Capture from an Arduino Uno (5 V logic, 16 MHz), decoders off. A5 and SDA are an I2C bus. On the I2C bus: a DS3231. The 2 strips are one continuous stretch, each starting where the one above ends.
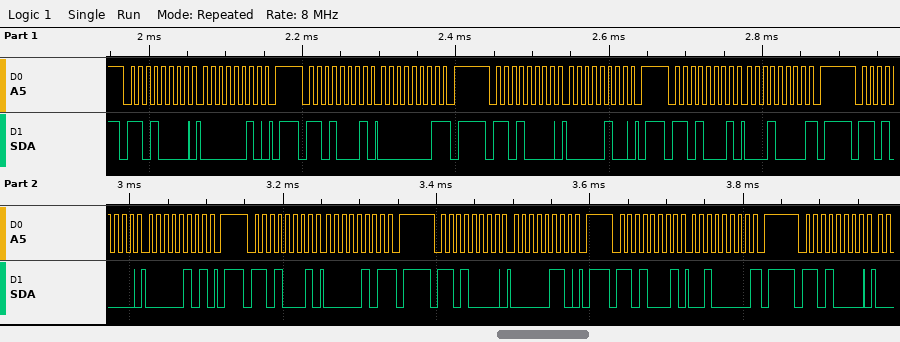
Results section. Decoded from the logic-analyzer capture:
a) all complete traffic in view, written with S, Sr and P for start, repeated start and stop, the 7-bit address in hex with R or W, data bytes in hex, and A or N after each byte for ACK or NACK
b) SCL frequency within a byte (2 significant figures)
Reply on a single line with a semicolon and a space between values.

S 68W A 02 A P S 68R A 01 N P S 68W A 04 A P S 68R A 10 N P S 68W A 05 A P S 68R A 05 N P S 68W A 06 A P S 68R A 20 N P S 68W A; 100 kHz
